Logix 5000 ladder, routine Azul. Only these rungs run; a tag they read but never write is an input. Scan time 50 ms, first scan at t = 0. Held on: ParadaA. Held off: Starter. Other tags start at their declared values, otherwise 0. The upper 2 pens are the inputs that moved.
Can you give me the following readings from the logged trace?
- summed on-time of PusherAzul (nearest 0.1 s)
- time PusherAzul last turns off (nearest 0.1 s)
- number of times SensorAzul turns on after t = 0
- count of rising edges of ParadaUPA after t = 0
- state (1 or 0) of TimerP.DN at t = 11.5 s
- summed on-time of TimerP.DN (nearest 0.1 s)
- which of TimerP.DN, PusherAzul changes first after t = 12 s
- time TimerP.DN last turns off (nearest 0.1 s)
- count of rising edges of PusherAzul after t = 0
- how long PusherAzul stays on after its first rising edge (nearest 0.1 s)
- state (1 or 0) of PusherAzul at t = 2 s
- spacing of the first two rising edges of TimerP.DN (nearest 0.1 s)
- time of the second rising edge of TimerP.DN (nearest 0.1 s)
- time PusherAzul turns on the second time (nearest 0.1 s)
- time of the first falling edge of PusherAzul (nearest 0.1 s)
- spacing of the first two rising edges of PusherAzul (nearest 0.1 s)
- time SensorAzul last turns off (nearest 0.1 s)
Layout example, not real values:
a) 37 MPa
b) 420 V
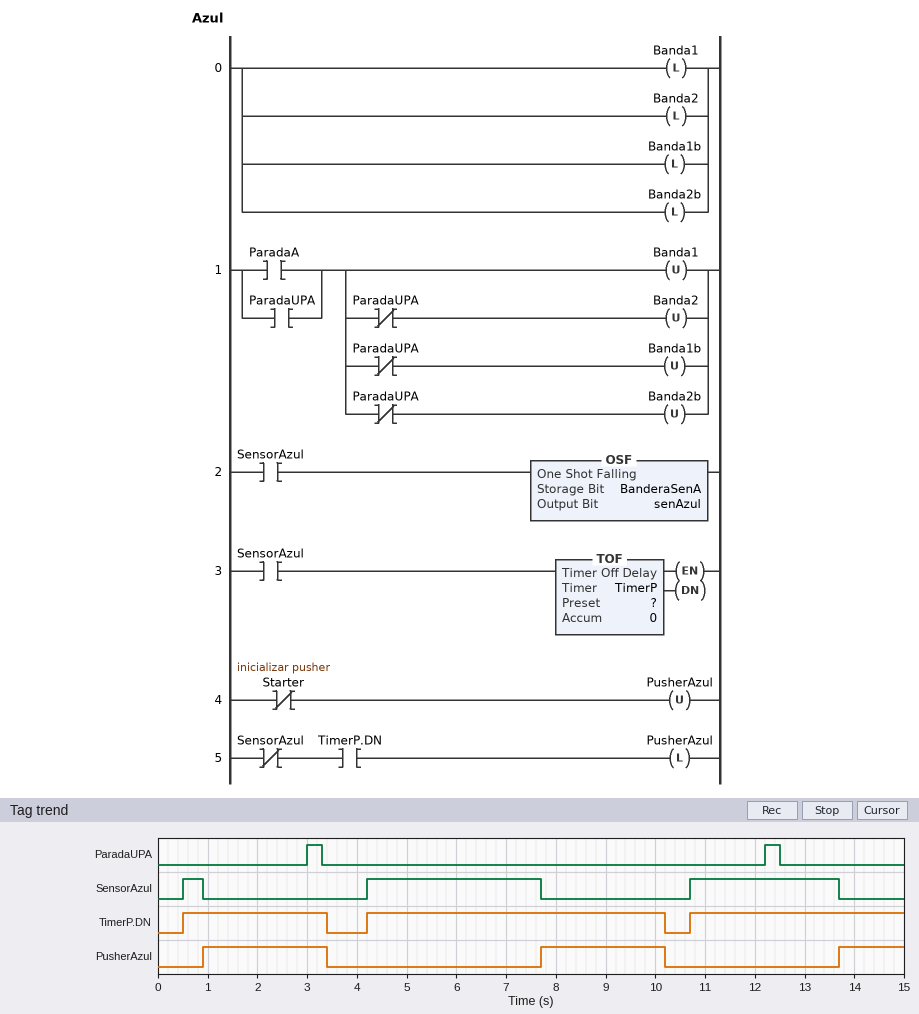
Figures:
a) 6.3 s
b) 10.2 s
c) 3
d) 2
e) 1
f) 13.2 s
g) PusherAzul
h) 10.2 s
i) 3
j) 2.5 s
k) 1
l) 3.7 s
m) 4.2 s
n) 7.7 s
o) 3.4 s
p) 6.8 s
q) 13.7 s
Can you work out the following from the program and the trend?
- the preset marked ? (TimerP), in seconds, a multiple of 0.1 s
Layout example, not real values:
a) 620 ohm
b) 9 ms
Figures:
a) 2.5 s
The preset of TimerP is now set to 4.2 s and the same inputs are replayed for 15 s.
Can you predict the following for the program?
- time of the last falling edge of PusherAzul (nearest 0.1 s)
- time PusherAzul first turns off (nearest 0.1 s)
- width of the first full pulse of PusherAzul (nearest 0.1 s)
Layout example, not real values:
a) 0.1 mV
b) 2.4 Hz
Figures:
a) 10.7 s
b) 4.2 s
c) 3.3 s
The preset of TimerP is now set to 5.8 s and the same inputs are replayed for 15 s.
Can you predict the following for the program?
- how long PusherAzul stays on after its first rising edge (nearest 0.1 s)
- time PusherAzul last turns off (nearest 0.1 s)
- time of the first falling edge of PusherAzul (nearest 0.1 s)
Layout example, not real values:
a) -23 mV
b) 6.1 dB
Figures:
a) 3.3 s
b) 10.7 s
c) 4.2 s
